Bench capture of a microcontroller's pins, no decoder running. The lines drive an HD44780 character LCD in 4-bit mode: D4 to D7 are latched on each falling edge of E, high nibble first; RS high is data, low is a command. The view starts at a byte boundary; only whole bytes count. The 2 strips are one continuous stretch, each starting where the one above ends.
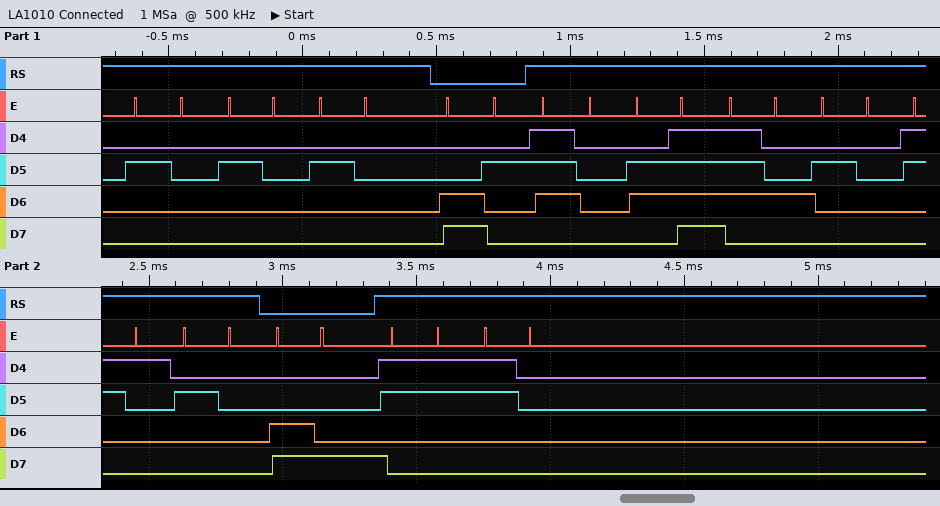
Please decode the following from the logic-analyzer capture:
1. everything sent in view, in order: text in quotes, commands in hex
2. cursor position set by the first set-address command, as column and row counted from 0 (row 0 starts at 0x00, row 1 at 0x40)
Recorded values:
"   " 0xC2 "pot 1 " 0xC8 "30"
column 2, row 1
